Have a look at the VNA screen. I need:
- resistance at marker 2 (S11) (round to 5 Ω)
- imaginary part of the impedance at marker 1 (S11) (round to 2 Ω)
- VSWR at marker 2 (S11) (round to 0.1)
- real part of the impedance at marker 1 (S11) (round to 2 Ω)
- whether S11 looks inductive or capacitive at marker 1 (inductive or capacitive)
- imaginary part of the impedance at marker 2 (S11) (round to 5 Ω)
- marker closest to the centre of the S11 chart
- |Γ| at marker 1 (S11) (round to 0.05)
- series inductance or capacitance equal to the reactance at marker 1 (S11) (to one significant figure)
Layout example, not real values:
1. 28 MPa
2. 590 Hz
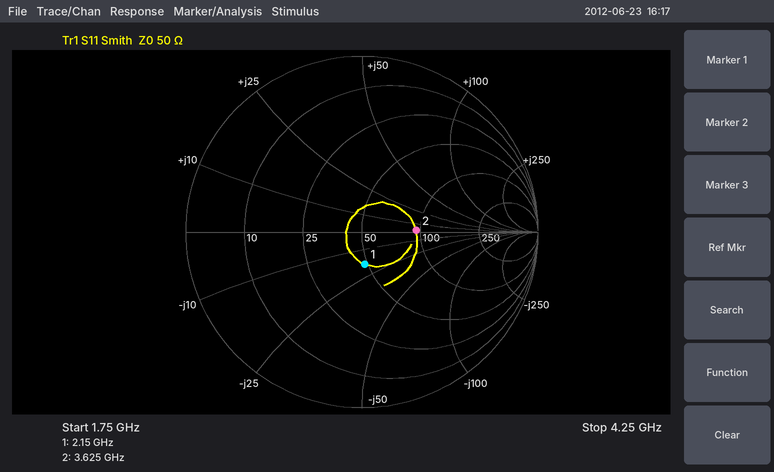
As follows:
1. 95 Ω
2. -18 Ω
3. 1.9
4. 48 Ω
5. capacitive
6. 0 Ω
7. marker 1
8. 0.20
9. 4 pF
